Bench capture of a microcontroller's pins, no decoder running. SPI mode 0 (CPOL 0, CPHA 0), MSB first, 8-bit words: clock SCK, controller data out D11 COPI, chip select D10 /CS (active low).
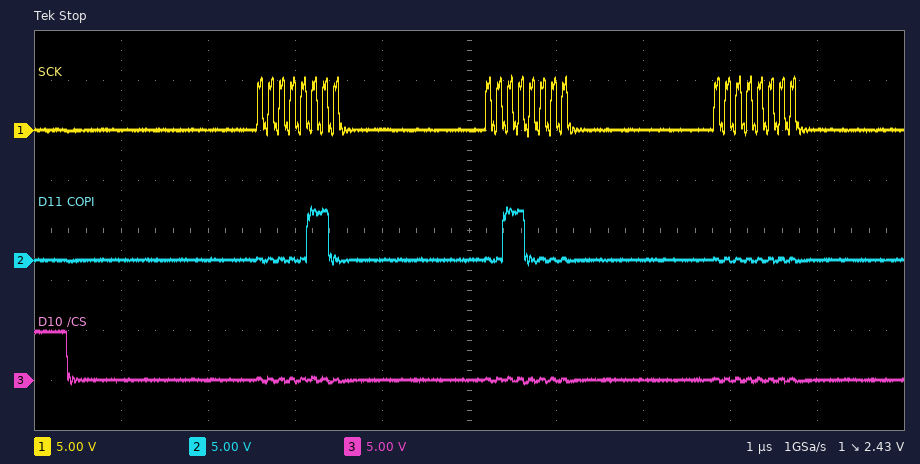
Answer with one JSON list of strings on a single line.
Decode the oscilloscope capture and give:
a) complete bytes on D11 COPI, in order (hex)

["06 30 00"]
